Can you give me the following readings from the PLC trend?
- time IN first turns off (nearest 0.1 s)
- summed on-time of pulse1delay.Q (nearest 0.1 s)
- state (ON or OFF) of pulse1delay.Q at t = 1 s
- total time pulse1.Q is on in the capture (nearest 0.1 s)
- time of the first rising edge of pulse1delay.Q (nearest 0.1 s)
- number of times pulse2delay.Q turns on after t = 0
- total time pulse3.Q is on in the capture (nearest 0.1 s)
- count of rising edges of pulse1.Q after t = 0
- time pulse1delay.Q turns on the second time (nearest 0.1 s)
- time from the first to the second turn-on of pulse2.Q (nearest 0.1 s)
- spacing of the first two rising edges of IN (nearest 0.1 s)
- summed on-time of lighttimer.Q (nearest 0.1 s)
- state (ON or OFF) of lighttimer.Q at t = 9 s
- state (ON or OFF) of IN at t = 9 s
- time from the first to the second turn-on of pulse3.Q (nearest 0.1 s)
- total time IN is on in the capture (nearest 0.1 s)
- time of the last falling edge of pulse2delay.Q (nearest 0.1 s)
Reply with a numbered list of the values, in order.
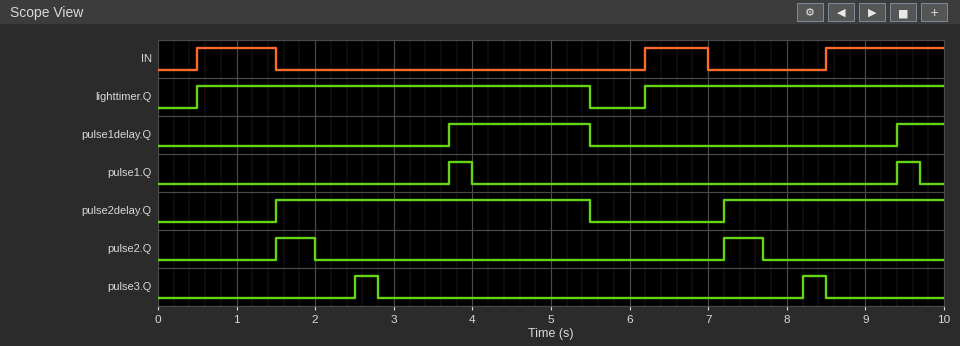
1. 1.5 s
2. 2.4 s
3. OFF
4. 0.6 s
5. 3.7 s
6. 2
7. 0.6 s
8. 2
9. 9.4 s
10. 5.7 s
11. 5.7 s
12. 8.8 s
13. ON
14. ON
15. 5.7 s
16. 3.3 s
17. 5.5 s
